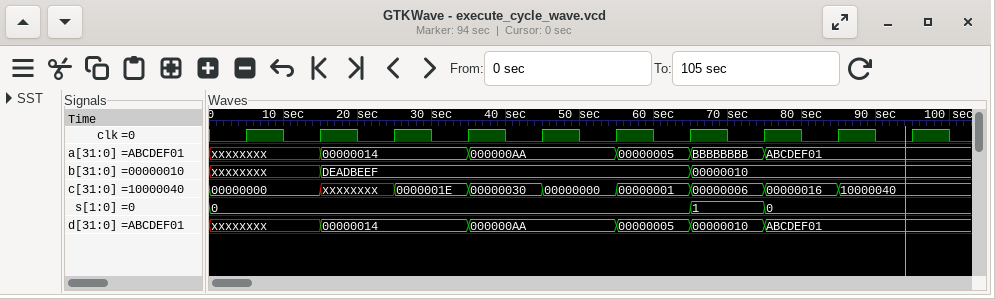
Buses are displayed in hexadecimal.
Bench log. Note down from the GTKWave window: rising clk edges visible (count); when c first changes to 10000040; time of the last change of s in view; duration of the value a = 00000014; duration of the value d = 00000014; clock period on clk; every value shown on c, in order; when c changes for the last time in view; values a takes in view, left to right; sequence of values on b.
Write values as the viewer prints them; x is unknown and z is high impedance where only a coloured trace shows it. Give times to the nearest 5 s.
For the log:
10
85 s
75 s
20 s
20 s
10 s
00000000, xxxxxxxx, 0000001E, 00000030, 00000000, 00000001, 00000006, 00000016, 10000040
85 s
xxxxxxxx, 00000014, 000000AA, 00000005, BBBBBBBB, ABCDEF01
xxxxxxxx, DEADBEEF, 00000010
